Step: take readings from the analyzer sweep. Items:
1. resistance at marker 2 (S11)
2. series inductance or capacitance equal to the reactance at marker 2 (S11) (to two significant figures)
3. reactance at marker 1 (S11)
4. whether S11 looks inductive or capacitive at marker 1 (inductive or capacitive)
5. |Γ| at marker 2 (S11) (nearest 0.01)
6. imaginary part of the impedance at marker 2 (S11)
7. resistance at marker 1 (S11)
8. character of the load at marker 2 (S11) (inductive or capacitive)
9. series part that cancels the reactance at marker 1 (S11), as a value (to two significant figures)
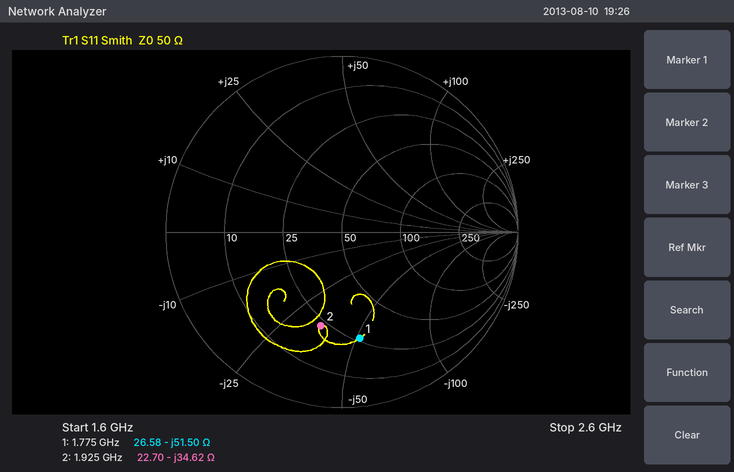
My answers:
22.70 Ω
2.4 pF
-51.50 Ω
capacitive
0.55
-34.62 Ω
26.58 Ω
capacitive
4.6 nH
